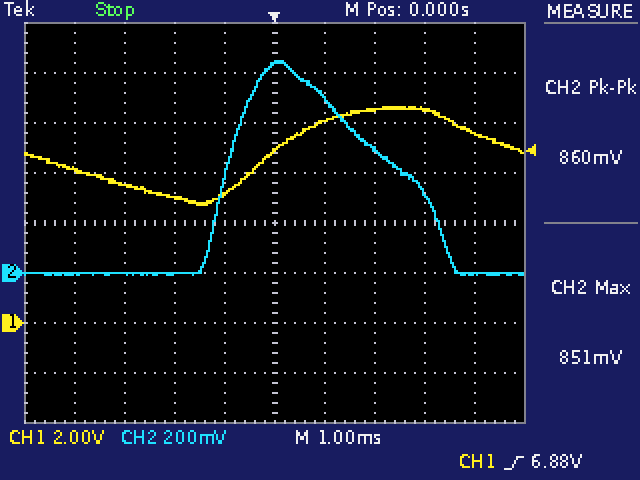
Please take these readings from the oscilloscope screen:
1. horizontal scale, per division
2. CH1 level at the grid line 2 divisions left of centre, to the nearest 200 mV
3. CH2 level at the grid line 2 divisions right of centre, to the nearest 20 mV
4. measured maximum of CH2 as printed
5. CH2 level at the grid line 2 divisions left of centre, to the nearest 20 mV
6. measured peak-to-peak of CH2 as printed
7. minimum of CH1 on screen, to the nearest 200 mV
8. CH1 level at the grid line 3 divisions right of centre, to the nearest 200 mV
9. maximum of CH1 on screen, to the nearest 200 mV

1 ms
5.0 V
500 mV
851 mV
0 mV
860 mV
4.8 V
8.6 V
8.6 V
